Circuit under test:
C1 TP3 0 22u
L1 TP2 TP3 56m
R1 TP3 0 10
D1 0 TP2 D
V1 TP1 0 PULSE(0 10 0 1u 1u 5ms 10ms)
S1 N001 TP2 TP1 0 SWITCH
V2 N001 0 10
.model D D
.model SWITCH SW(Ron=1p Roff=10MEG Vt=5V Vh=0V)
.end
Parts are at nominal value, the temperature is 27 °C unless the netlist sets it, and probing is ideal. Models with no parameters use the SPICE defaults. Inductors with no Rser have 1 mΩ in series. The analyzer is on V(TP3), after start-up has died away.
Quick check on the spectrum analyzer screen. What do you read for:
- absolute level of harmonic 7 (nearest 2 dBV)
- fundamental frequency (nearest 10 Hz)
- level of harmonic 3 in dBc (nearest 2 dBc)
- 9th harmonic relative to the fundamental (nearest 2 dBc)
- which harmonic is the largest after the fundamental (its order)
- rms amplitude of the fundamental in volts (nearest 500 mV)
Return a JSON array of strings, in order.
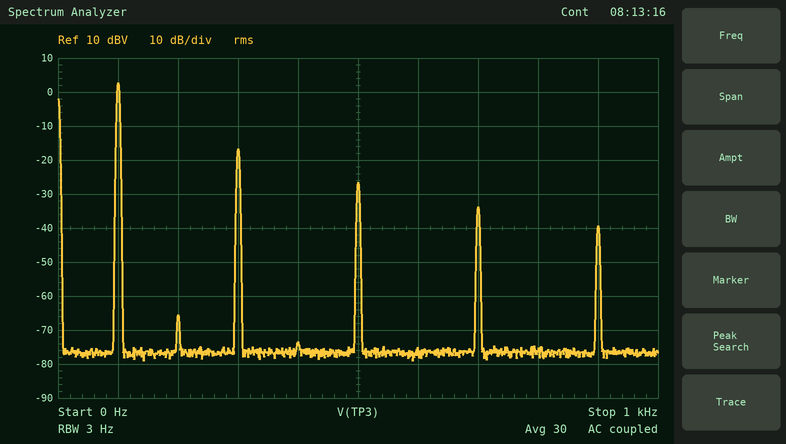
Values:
["-34 dBV", "100 Hz", "-20 dBc", "-42 dBc", "3", "1.5 V"]
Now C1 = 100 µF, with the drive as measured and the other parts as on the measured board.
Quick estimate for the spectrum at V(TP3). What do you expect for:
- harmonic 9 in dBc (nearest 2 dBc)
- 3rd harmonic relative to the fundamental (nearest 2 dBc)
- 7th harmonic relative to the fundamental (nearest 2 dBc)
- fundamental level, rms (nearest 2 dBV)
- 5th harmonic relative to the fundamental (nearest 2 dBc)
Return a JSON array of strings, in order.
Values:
["-52 dBc", "-24 dBc", "-46 dBc", "2 dBV", "-38 dBc"]
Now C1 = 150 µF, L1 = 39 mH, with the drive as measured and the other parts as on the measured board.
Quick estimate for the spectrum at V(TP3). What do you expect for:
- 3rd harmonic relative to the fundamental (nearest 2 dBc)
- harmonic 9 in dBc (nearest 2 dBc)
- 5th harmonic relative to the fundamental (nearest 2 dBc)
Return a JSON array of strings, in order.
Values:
["-28 dBc", "-56 dBc", "-40 dBc"]
